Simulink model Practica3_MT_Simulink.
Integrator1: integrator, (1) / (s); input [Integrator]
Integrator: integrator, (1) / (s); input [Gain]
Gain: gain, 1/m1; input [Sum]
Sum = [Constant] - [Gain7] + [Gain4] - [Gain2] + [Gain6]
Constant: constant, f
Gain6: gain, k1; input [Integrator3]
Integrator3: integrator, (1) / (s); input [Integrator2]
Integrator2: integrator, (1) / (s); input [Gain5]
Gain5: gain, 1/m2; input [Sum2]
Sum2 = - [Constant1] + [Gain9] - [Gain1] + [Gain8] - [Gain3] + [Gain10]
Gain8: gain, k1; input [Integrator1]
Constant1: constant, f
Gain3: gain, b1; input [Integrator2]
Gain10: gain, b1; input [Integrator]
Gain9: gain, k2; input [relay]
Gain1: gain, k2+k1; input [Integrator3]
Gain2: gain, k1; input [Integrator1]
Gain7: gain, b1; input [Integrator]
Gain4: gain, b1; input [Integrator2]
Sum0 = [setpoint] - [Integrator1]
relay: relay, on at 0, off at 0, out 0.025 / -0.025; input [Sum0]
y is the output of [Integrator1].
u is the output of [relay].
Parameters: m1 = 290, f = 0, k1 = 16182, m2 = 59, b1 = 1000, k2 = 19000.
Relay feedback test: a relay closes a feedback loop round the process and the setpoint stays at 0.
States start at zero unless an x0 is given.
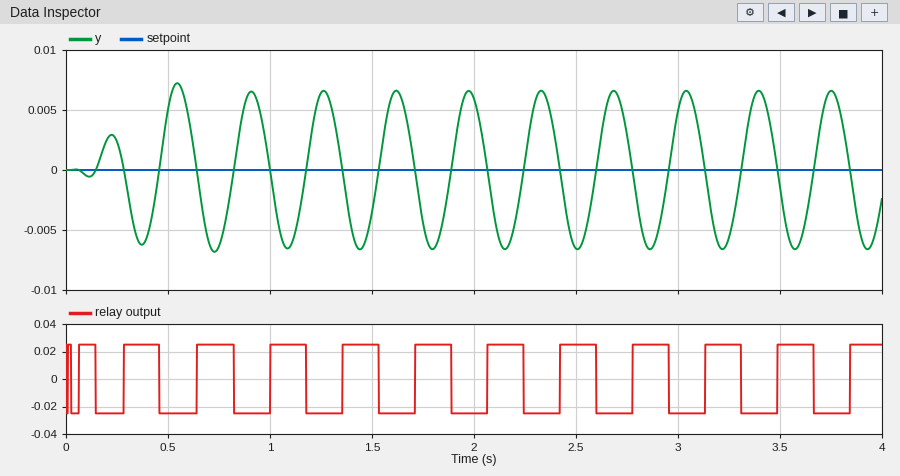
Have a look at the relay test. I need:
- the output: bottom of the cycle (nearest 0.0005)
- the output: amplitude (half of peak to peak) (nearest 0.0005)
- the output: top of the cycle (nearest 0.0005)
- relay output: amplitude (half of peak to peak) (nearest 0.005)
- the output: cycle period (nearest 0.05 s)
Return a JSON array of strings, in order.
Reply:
["-0.0065", "0.0065", "0.0065", "0.025", "0.35 s"]
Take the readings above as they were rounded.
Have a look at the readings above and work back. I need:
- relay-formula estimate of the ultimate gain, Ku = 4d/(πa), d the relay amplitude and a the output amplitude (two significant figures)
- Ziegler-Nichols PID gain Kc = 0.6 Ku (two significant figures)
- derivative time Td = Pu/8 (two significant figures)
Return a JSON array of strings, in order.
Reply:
["4.9", "2.9", "0.044 s"]
